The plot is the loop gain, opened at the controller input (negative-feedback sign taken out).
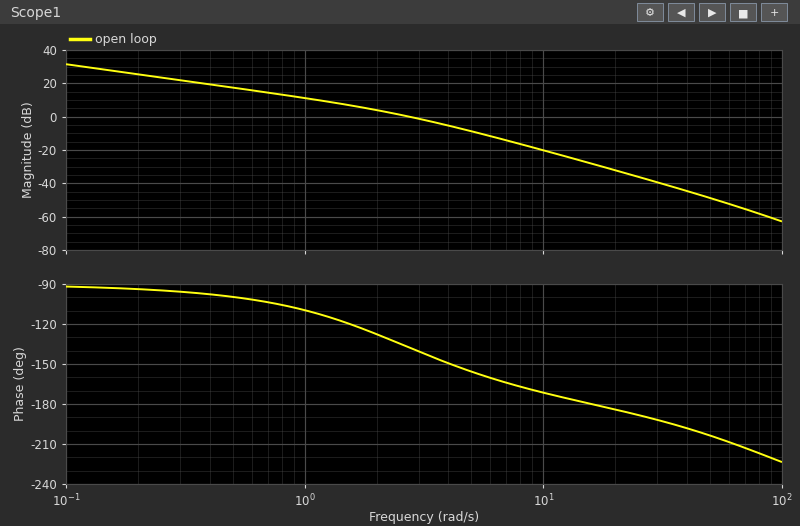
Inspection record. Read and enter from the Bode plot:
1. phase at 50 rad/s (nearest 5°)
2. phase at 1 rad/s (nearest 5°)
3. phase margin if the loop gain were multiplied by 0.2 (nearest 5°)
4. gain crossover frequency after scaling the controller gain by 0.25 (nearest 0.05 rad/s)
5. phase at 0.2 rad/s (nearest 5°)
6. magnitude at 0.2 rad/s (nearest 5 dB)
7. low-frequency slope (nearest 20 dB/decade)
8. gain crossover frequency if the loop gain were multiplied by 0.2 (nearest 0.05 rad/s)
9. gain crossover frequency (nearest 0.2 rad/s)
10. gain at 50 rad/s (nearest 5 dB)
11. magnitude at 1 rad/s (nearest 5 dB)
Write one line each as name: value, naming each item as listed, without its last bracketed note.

phase at 50 rad/s: -205°
phase at 1 rad/s: -110°
phase margin if the loop gain were multiplied by 0.2: 75°
gain crossover frequency after scaling the controller gain by 0.25: 0.90 rad/s
phase at 0.2 rad/s: -95°
magnitude at 0.2 rad/s: 25 dB
low-frequency slope: -20 dB/decade
gain crossover frequency if the loop gain were multiplied by 0.2: 0.75 rad/s
gain crossover frequency: 2.8 rad/s
gain at 50 rad/s: -50 dB
magnitude at 1 rad/s: 10 dB
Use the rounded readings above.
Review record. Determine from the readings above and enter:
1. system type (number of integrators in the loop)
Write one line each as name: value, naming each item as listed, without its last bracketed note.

system type: 1
